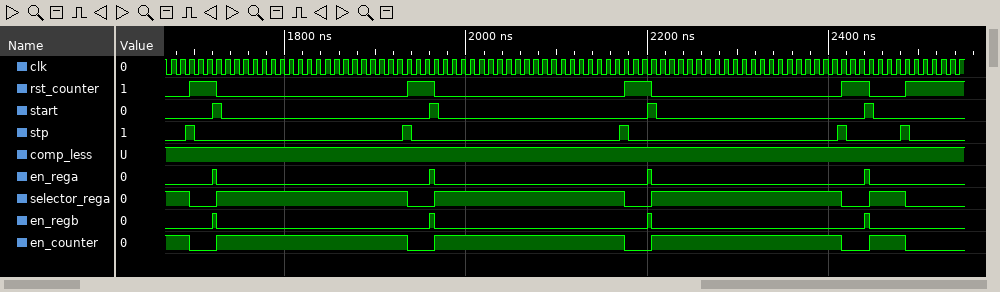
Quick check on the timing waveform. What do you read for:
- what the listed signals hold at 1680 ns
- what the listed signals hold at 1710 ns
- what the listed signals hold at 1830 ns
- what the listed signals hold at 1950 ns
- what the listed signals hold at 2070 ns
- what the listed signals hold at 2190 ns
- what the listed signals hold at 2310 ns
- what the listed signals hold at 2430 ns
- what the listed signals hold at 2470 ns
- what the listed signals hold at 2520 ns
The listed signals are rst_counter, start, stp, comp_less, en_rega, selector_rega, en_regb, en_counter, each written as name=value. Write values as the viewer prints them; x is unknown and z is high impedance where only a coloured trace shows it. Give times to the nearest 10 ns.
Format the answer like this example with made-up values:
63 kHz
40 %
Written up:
rst_counter=0, start=0, stp=0, comp_less=1, en_rega=0, selector_rega=1, en_regb=0, en_counter=1
rst_counter=1, start=0, stp=0, comp_less=1, en_rega=0, selector_rega=0, en_regb=0, en_counter=0
rst_counter=0, start=0, stp=0, comp_less=1, en_rega=0, selector_rega=1, en_regb=0, en_counter=1
rst_counter=1, start=0, stp=0, comp_less=1, en_rega=0, selector_rega=0, en_regb=0, en_counter=0
rst_counter=0, start=0, stp=0, comp_less=1, en_rega=0, selector_rega=1, en_regb=0, en_counter=1
rst_counter=1, start=0, stp=0, comp_less=1, en_rega=0, selector_rega=0, en_regb=0, en_counter=0
rst_counter=0, start=0, stp=0, comp_less=1, en_rega=0, selector_rega=1, en_regb=0, en_counter=1
rst_counter=1, start=0, stp=0, comp_less=1, en_rega=0, selector_rega=0, en_regb=0, en_counter=0
rst_counter=0, start=0, stp=0, comp_less=1, en_rega=0, selector_rega=1, en_regb=0, en_counter=1
rst_counter=1, start=0, stp=0, comp_less=1, en_rega=0, selector_rega=0, en_regb=0, en_counter=0
